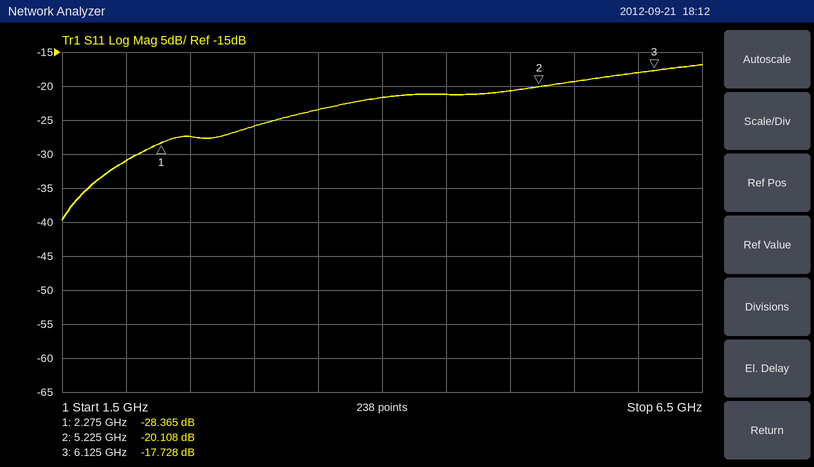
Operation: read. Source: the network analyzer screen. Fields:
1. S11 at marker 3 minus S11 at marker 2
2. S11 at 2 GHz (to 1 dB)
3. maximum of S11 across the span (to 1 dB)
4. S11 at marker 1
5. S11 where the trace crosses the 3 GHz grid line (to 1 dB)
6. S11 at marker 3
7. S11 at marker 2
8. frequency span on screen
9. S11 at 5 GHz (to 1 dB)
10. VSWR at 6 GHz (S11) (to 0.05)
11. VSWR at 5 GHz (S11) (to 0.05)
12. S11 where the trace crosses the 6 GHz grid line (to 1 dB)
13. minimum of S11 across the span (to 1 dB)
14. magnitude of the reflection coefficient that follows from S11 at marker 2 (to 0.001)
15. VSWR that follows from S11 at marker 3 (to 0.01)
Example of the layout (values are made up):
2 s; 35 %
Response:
2.380 dB; -31 dB; -17 dB; -28.365 dB; -26 dB; -17.728 dB; -20.108 dB; 5 GHz; -21 dB; 1.30; 1.20; -18 dB; -40 dB; 0.099; 1.30
